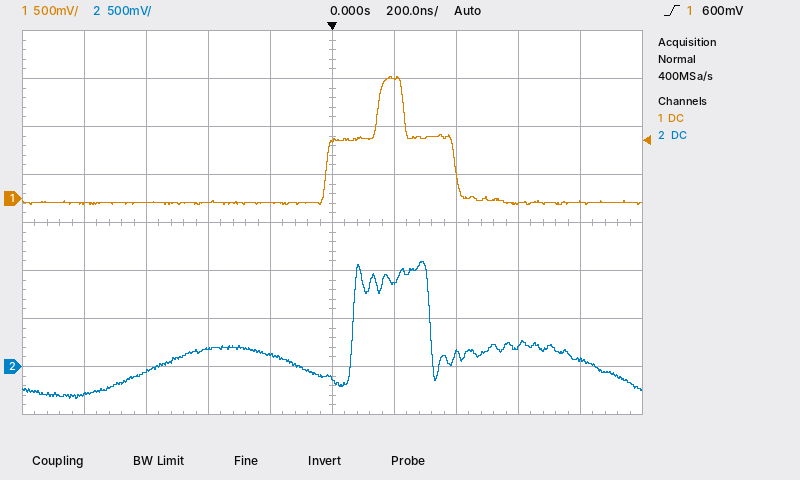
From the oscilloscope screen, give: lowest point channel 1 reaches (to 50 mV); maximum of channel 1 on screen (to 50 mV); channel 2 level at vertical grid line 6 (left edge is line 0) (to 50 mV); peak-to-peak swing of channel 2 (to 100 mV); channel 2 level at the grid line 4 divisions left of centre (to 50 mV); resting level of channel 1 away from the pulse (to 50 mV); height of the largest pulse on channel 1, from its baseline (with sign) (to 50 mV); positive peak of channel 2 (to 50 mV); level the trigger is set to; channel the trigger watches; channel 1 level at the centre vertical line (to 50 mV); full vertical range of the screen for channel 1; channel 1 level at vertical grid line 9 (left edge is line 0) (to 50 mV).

-50 mV
1.25 V
900 mV
1.40 V
-300 mV
-50 mV
+1.30 V
1.10 V
600 mV
channel 1
600 mV
4 V
-50 mV
